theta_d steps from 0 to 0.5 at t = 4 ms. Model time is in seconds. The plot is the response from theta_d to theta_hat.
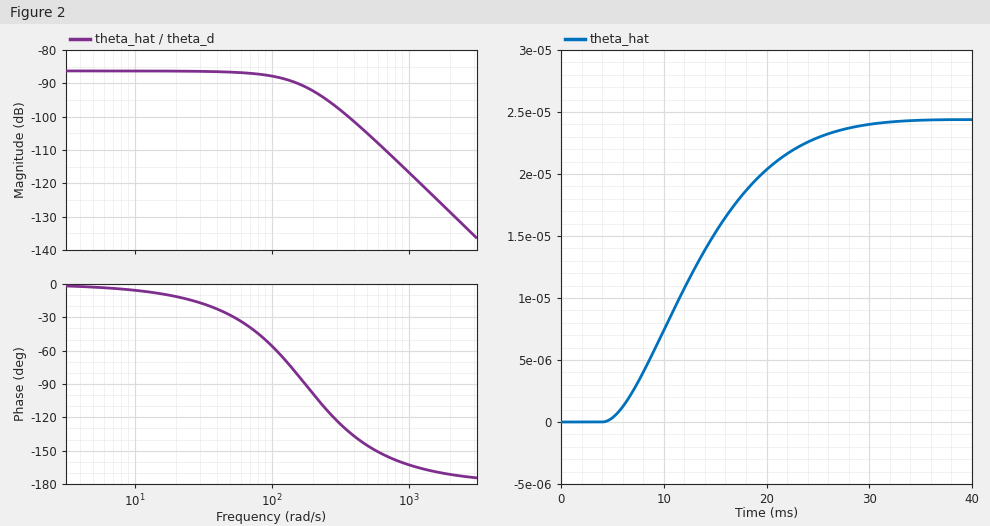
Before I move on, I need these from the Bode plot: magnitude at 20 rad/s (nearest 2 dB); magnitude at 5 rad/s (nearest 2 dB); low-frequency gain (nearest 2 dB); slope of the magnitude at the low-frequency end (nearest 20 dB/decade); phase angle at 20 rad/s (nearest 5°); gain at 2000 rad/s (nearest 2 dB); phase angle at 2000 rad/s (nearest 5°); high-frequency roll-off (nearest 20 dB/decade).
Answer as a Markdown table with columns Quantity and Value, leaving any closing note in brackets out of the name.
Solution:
| Quantity | Value |
|---|---|
| magnitude at 20 rad/s | -86 dB |
| magnitude at 5 rad/s | -86 dB |
| low-frequency gain | -86 dB |
| slope of the magnitude at the low-frequency end | 0 dB/decade |
| phase angle at 20 rad/s | -10° |
| gain at 2000 rad/s | -128 dB |
| phase angle at 2000 rad/s | -170° |
| high-frequency roll-off | -40 dB/decade |
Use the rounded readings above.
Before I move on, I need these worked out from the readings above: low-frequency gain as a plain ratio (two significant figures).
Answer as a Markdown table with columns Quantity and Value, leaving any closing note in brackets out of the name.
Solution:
| Quantity | Value |
|---|---|
| low-frequency gain as a plain ratio | 0.000050 |
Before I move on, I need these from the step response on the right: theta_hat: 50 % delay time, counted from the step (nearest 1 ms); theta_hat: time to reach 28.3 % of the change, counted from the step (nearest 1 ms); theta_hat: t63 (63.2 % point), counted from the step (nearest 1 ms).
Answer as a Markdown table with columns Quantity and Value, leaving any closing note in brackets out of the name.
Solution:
| Quantity | Value |
|---|---|
| theta_hat: 50 % delay time, counted from the step | 9 ms |
| theta_hat: time to reach 28.3 % of the change, counted from the step | 6 ms |
| theta_hat: t63 (63.2 % point), counted from the step | 11 ms |
